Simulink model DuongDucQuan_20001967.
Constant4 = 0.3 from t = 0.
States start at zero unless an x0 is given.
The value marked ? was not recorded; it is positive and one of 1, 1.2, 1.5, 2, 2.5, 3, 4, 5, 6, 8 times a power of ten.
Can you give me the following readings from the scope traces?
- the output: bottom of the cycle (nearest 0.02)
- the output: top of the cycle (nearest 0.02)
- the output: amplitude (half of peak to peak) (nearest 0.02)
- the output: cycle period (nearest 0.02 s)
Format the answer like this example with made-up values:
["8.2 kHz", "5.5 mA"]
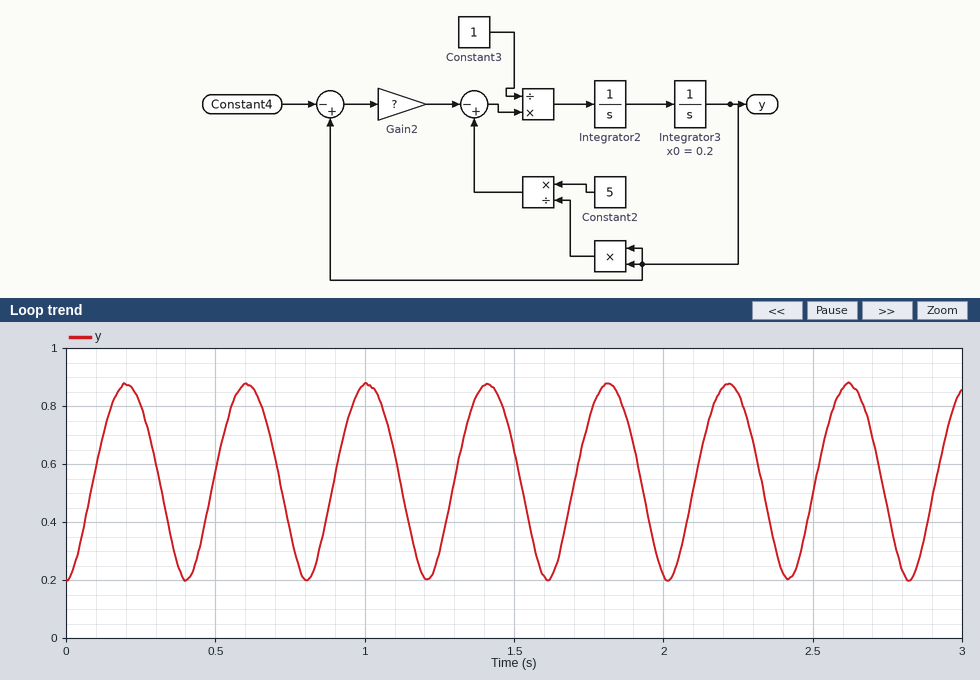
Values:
["0.20", "0.88", "0.34", "0.40 s"]
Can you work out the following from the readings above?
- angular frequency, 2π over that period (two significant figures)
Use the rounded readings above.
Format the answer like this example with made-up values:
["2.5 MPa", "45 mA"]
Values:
["16 rad/s"]
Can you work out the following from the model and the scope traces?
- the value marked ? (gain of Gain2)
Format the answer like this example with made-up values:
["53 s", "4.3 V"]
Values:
["120"]
